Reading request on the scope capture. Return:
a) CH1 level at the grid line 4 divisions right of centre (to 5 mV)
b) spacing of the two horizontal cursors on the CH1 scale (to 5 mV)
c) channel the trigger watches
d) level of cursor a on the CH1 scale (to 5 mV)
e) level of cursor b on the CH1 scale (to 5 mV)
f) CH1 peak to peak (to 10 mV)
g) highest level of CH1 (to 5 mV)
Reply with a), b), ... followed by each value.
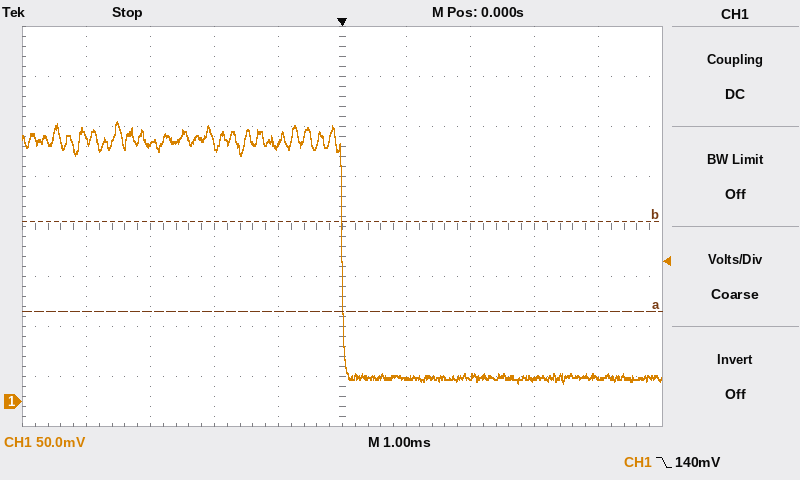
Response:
a) 25 mV
b) 90 mV
c) CH1
d) 90 mV
e) 180 mV
f) 260 mV
g) 280 mV
